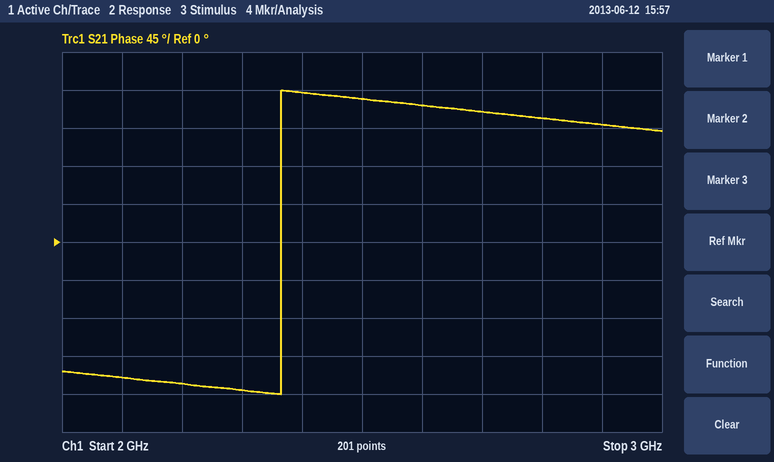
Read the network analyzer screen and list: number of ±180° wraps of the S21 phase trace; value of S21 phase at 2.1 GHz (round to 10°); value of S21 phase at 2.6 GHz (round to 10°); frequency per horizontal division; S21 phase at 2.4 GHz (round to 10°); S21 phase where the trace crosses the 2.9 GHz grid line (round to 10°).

1
-160°
160°
100 MHz
180°
140°
